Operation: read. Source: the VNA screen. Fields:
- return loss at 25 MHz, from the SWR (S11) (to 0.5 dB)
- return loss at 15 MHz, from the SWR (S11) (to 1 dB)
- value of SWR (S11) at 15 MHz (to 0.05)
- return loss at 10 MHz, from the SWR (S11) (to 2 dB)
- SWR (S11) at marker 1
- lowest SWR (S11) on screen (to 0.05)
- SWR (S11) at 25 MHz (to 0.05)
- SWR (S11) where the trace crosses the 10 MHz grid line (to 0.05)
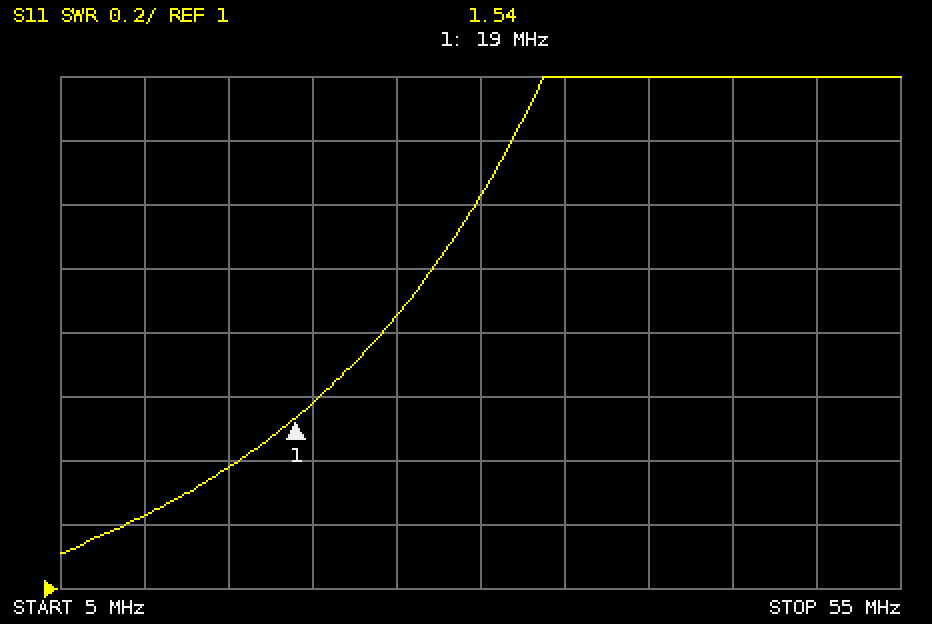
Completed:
10.5 dB
16 dB
1.40
20 dB
1.54
1.10
1.85
1.25
